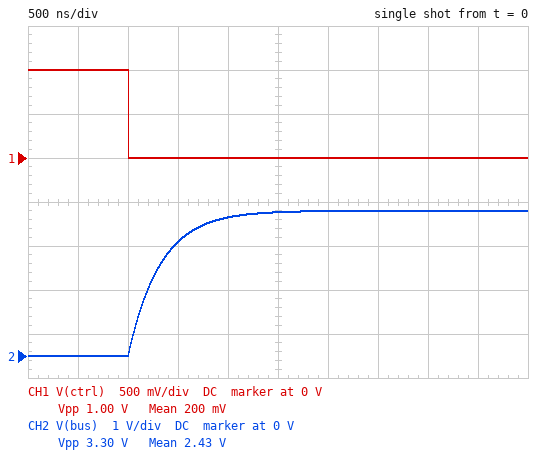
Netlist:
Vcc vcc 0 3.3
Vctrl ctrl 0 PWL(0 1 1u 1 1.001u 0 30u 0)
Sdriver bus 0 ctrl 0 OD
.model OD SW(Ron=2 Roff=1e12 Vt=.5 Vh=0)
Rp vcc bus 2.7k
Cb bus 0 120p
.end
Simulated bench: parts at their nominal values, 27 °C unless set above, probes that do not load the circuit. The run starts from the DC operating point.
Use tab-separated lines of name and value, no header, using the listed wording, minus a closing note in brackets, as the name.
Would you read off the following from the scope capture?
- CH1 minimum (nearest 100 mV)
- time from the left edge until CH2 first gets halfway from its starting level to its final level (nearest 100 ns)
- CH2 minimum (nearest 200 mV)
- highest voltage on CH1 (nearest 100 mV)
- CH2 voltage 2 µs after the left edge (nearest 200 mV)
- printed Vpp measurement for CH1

CH1 minimum	0 V
time from the left edge until CH2 first gets halfway from its starting level to its final level	1.2 µs
CH2 minimum	0 V
highest voltage on CH1	1.0 V
CH2 voltage 2 µs after the left edge	3.2 V
printed Vpp measurement for CH1	1.00 V
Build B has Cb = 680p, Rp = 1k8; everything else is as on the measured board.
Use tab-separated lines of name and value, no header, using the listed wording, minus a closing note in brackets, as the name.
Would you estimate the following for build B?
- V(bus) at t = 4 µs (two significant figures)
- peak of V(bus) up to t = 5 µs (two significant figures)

V(bus) at t = 4 µs	3.0 V
peak of V(bus) up to t = 5 µs	3.2 V
